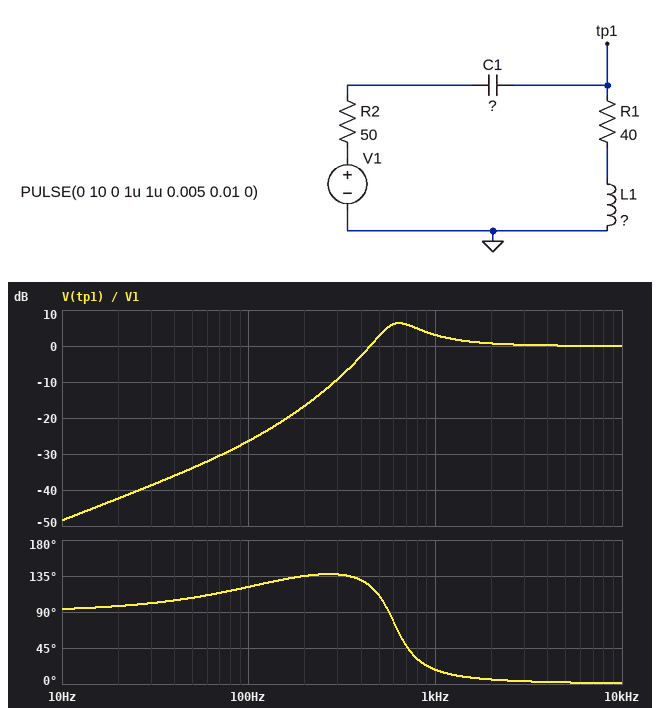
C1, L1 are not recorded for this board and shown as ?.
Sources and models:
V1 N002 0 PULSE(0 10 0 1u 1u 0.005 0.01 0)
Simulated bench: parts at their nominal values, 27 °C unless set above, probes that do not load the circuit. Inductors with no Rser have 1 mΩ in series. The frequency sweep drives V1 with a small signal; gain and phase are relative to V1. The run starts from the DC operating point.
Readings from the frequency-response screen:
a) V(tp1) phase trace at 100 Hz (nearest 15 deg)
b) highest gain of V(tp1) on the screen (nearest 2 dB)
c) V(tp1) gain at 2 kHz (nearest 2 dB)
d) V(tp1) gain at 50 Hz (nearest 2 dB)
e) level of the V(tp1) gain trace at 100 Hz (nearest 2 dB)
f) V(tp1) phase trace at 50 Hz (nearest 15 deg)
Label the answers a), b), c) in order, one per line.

a) 120 deg
b) 6 dB
c) 0 dB
d) -34 dB
e) -26 dB
f) 105 deg
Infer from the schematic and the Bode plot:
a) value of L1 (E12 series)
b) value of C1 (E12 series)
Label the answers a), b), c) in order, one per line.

a) 47 mH
b) 1.5 µF
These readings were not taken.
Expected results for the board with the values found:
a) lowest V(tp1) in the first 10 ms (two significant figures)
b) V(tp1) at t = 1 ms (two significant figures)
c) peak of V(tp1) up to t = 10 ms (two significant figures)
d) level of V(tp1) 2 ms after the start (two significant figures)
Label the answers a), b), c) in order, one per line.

a) -9.9 V
b) -3.3 V
c) 10 V
d) 760 mV
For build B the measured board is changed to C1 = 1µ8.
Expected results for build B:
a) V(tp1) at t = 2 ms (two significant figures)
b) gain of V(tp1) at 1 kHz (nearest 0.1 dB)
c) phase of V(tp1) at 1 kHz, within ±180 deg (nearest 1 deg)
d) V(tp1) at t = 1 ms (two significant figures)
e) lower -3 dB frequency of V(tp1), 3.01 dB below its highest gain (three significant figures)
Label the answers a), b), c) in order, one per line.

a) 1.4 V
b) 2.4 dB
c) 16 deg
d) -3.8 V
e) 463 Hz
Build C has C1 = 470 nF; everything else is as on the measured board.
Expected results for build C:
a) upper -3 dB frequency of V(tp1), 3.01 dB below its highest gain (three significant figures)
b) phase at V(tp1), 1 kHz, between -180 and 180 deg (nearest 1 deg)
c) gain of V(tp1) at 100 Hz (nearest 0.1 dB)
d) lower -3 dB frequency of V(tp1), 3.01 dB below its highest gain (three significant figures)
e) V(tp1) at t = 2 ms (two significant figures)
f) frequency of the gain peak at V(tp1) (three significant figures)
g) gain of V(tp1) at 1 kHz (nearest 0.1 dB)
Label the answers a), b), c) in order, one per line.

a) 1.30 kHz
b) 108 deg
c) -36.6 dB
d) 961 Hz
e) 1.1 V
f) 1.09 kHz
g) 9.5 dB
